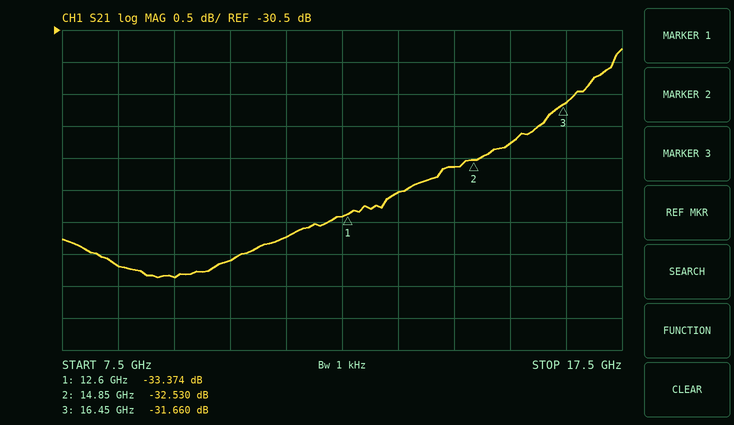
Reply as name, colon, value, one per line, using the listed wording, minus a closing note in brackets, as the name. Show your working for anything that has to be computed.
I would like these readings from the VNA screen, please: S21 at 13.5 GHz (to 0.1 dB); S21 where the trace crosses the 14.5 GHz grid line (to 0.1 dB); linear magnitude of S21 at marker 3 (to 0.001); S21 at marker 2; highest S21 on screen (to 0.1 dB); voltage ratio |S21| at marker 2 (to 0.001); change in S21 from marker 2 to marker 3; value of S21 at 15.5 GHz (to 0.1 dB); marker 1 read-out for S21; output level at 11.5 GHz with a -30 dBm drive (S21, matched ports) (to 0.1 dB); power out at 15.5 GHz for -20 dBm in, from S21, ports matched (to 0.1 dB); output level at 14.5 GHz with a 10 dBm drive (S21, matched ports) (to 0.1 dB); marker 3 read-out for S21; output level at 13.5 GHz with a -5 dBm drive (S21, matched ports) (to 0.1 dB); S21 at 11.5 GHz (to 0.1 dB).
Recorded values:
S21 at 13.5 GHz: -33.0 dB
S21 where the trace crosses the 14.5 GHz grid line: -32.6 dB
linear magnitude of S21 at marker 3: 10^(-31.66/20) ≈ 0.026
S21 at marker 2: -32.530 dB
highest S21 on screen: -30.8 dB
voltage ratio |S21| at marker 2: 10^(-32.53/20) ≈ 0.024
change in S21 from marker 2 to marker 3: -31.66 − (-32.53) = 0.870 dB
value of S21 at 15.5 GHz: -32.3 dB
marker 1 read-out for S21: -33.374 dB
output level at 11.5 GHz with a -30 dBm drive (S21, matched ports): -30 dBm + (-33.7 dB) = -63.7 dBm
power out at 15.5 GHz for -20 dBm in, from S21, ports matched: -20 dBm + (-32.3 dB) = -52.3 dBm
output level at 14.5 GHz with a 10 dBm drive (S21, matched ports): 10 dBm + (-32.6 dB) = -22.6 dBm
marker 3 read-out for S21: -31.660 dB
output level at 13.5 GHz with a -5 dBm drive (S21, matched ports): -5 dBm + (-33.0 dB) = -38.0 dBm
S21 at 11.5 GHz: -33.7 dB
